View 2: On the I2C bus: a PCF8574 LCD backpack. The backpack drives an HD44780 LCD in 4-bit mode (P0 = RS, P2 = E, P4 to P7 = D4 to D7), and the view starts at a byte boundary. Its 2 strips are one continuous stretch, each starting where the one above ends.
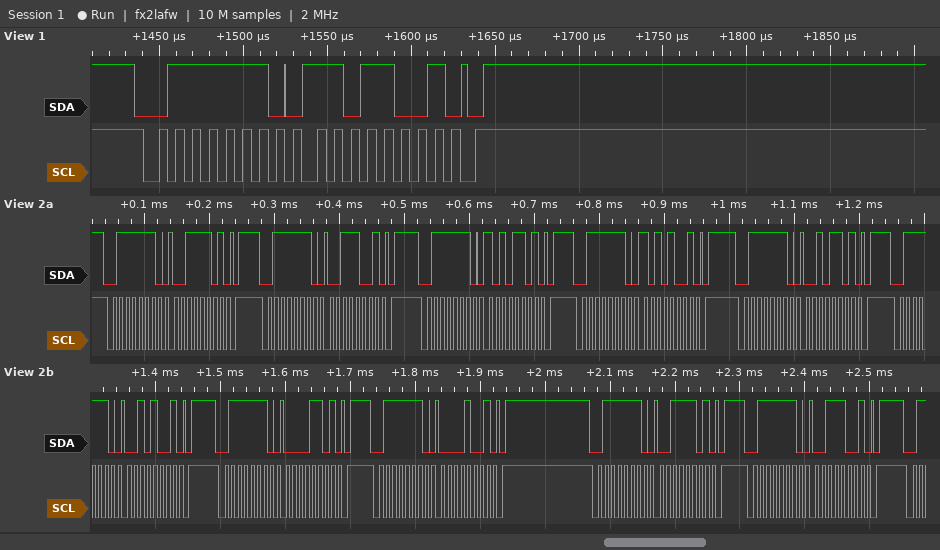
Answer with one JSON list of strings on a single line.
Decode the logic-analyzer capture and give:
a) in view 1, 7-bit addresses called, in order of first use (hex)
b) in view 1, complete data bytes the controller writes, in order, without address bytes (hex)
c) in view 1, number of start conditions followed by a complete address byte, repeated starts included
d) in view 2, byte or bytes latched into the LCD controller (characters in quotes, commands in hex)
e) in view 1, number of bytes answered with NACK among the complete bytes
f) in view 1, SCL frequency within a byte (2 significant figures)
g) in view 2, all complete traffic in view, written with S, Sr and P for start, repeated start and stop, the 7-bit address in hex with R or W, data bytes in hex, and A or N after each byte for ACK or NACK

["0x3F", "D9", "1", "':' ' '", "0", "100 kHz", "S 3FW A 3D A P S 3FW A 39 A P S 3FW A AD A P S 3FW A A9 A P S 3FW A 2D A P S 3FW A 29 A P S 3FW A 0D A P S 3FW A 09 A P S 3FW A 3D A P S 3FW A 39 A P"]
